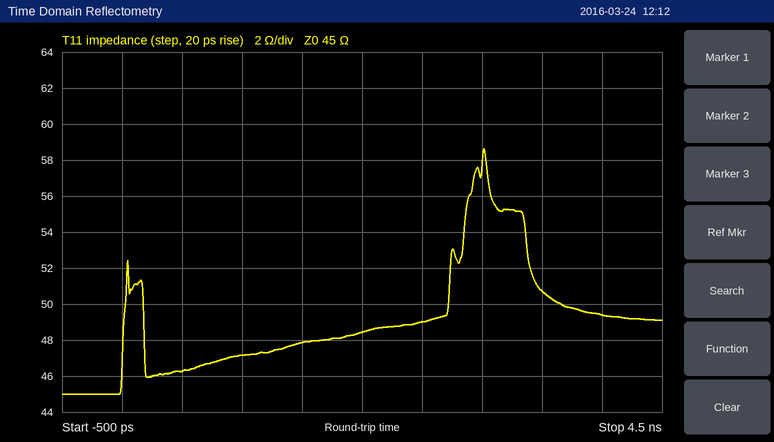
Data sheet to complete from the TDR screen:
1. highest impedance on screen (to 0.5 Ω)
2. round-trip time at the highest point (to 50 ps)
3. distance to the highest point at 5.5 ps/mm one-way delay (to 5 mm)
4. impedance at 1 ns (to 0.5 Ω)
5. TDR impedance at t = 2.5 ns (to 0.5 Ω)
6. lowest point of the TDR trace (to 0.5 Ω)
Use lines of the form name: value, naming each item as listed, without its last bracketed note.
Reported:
highest impedance on screen: 58.5 Ω
round-trip time at the highest point: 3.00 ns
distance to the highest point at 5.5 ps/mm one-way delay: 275 mm
impedance at 1 ns: 47.0 Ω
TDR impedance at t = 2.5 ns: 49.0 Ω
lowest point of the TDR trace: 45.0 Ω
